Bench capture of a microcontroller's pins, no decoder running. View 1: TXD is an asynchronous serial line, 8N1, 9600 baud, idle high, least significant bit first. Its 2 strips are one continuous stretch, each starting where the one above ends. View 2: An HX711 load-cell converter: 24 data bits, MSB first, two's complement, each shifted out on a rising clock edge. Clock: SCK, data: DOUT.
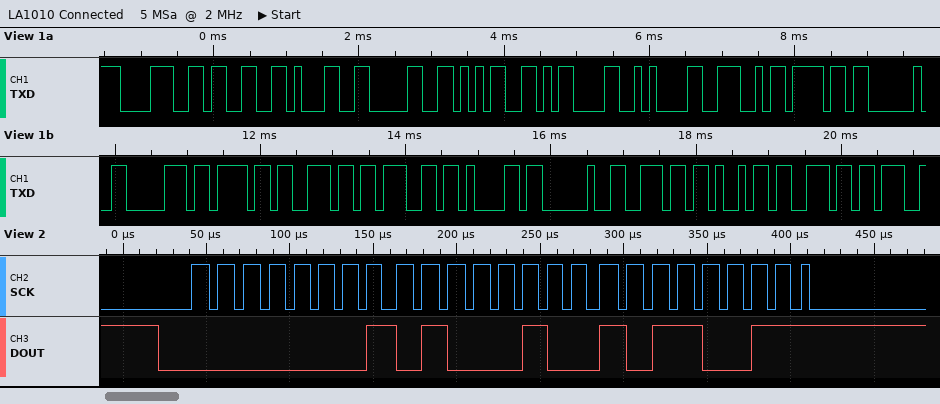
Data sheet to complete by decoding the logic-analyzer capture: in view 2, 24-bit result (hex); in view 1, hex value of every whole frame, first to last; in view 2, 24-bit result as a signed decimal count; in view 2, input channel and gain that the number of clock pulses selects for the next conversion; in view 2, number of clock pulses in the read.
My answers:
0x0144B3
38 33 31 30 35 0D 0A 4E 6F 20 70 6F 6E 67 61 20 6E 69 6E
83123
channel A, gain 128
25
